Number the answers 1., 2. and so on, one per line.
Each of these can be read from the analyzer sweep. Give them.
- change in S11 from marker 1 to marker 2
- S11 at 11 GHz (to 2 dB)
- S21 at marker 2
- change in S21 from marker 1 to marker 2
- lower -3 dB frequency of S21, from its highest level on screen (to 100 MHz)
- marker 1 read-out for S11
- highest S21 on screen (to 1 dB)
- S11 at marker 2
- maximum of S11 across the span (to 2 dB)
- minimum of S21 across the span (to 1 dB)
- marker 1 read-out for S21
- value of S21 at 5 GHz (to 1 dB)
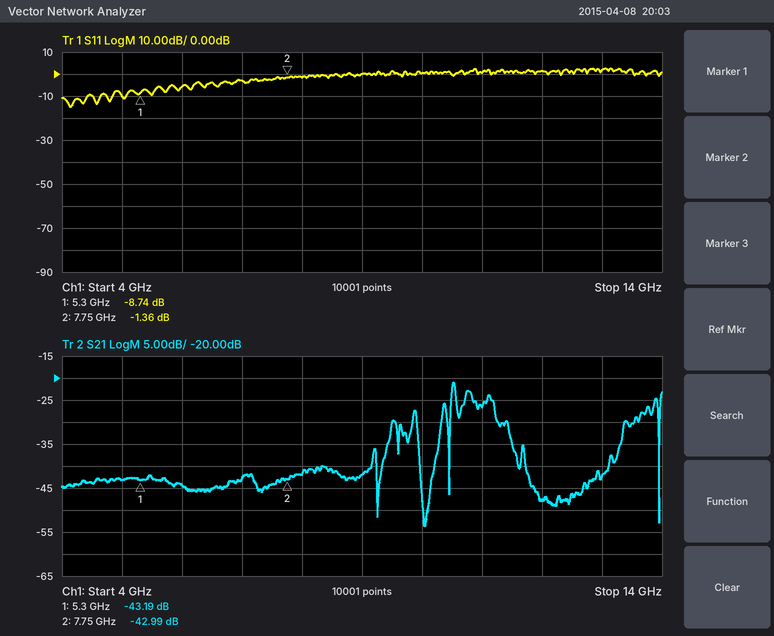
1. 7.38 dB
2. 0 dB
3. -42.99 dB
4. 0.20 dB
5. 10.5 GHz
6. -8.74 dB
7. -21 dB
8. -1.36 dB
9. 2 dB
10. -54 dB
11. -43.19 dB
12. -43 dB
